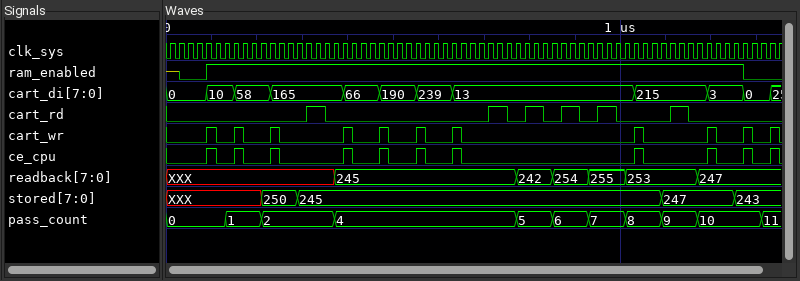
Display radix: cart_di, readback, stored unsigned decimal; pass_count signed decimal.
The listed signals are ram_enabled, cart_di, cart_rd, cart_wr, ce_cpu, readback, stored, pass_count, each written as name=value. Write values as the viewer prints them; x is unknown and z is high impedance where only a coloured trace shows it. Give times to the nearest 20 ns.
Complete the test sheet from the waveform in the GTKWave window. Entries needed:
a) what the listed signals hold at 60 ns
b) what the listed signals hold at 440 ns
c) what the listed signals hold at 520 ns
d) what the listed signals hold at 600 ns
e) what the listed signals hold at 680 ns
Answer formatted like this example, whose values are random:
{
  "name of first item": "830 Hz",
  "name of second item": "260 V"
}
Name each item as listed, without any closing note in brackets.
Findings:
{
  "what the listed signals hold at 60 ns": "ram_enabled=0, cart_di=0, cart_rd=0, cart_wr=0, ce_cpu=0, readback=XXX, stored=XXX, pass_count=0",
  "what the listed signals hold at 440 ns": "ram_enabled=1, cart_di=66, cart_rd=0, cart_wr=0, ce_cpu=0, readback=245, stored=245, pass_count=4",
  "what the listed signals hold at 520 ns": "ram_enabled=1, cart_di=190, cart_rd=0, cart_wr=0, ce_cpu=0, readback=245, stored=245, pass_count=4",
  "what the listed signals hold at 600 ns": "ram_enabled=1, cart_di=239, cart_rd=0, cart_wr=0, ce_cpu=0, readback=245, stored=245, pass_count=4",
  "what the listed signals hold at 680 ns": "ram_enabled=1, cart_di=13, cart_rd=0, cart_wr=0, ce_cpu=0, readback=245, stored=245, pass_count=4"
}
